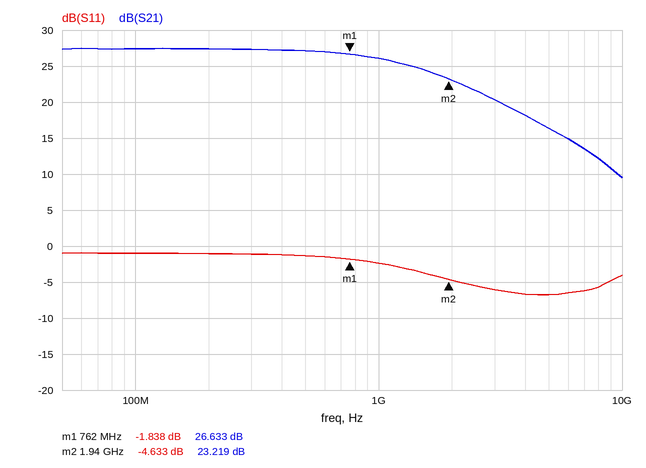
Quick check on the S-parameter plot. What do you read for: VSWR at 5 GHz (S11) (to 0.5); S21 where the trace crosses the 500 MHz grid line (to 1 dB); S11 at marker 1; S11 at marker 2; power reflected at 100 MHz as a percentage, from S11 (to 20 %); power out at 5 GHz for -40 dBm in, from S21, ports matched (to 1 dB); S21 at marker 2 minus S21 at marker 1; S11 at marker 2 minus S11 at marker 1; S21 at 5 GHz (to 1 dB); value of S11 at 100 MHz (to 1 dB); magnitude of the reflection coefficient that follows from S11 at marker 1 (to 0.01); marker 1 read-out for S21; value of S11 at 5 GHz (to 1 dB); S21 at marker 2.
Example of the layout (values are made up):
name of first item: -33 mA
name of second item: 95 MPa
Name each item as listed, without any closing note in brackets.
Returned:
VSWR at 5 GHz (S11): 2.5
S21 where the trace crosses the 500 MHz grid line: 27 dB
S11 at marker 1: -1.838 dB
S11 at marker 2: -4.633 dB
power reflected at 100 MHz as a percentage, from S11: 80 %
power out at 5 GHz for -40 dBm in, from S21, ports matched: -24 dBm
S21 at marker 2 minus S21 at marker 1: -3.414 dB
S11 at marker 2 minus S11 at marker 1: -2.795 dB
S21 at 5 GHz: 16 dB
value of S11 at 100 MHz: -1 dB
magnitude of the reflection coefficient that follows from S11 at marker 1: 0.81
marker 1 read-out for S21: 26.633 dB
value of S11 at 5 GHz: -7 dB
S21 at marker 2: 23.219 dB
